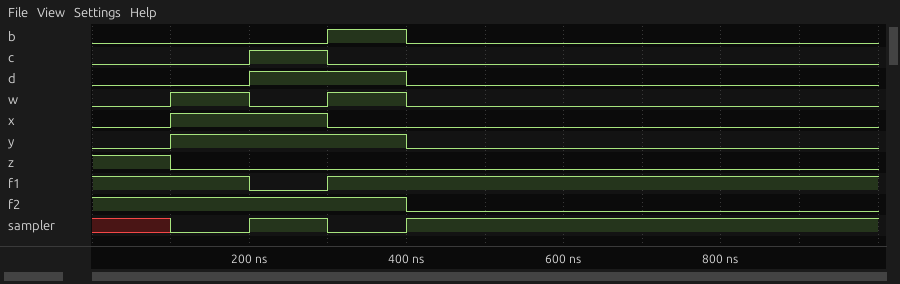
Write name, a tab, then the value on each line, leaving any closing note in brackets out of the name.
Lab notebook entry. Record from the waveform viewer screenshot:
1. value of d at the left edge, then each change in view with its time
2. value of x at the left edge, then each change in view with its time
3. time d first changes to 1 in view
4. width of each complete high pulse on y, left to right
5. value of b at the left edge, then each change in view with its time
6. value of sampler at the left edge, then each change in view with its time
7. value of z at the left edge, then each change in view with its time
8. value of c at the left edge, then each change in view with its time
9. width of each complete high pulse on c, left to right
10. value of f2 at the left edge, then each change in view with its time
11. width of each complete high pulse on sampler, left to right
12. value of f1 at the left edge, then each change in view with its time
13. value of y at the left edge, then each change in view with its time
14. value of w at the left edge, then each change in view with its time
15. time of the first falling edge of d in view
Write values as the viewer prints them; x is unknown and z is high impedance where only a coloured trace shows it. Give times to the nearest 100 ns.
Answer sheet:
value of d at the left edge, then each change in view with its time	0, 1 at 200 ns, 0 at 400 ns
value of x at the left edge, then each change in view with its time	0, 1 at 100 ns, 0 at 300 ns
time d first changes to 1 in view	200 ns
width of each complete high pulse on y, left to right	300 ns
value of b at the left edge, then each change in view with its time	0, 1 at 300 ns, 0 at 400 ns
value of sampler at the left edge, then each change in view with its time	x, 0 at 100 ns, 1 at 200 ns, 0 at 300 ns, 1 at 400 ns
value of z at the left edge, then each change in view with its time	1, 0 at 100 ns
value of c at the left edge, then each change in view with its time	0, 1 at 200 ns, 0 at 300 ns
width of each complete high pulse on c, left to right	100 ns
value of f2 at the left edge, then each change in view with its time	1, 0 at 400 ns
width of each complete high pulse on sampler, left to right	100 ns
value of f1 at the left edge, then each change in view with its time	1, 0 at 200 ns, 1 at 300 ns
value of y at the left edge, then each change in view with its time	0, 1 at 100 ns, 0 at 400 ns
value of w at the left edge, then each change in view with its time	0, 1 at 100 ns, 0 at 200 ns, 1 at 300 ns, 0 at 400 ns
time of the first falling edge of d in view	400 ns
